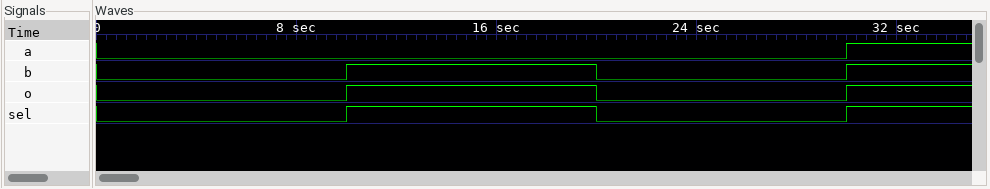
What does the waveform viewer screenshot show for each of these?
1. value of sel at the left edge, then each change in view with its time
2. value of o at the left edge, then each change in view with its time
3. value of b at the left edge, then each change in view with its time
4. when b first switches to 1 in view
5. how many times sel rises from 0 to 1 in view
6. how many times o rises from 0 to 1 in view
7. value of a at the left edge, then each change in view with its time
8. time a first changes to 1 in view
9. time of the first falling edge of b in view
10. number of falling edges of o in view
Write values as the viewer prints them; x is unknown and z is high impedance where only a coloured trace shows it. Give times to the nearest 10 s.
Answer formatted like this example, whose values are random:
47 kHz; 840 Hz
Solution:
0, 1 at 10 s, 0 at 20 s, 1 at 30 s; 0, 1 at 10 s, 0 at 20 s, 1 at 30 s; 0, 1 at 10 s, 0 at 20 s, 1 at 30 s; 10 s; 2; 2; 0, 1 at 30 s; 30 s; 20 s; 1
